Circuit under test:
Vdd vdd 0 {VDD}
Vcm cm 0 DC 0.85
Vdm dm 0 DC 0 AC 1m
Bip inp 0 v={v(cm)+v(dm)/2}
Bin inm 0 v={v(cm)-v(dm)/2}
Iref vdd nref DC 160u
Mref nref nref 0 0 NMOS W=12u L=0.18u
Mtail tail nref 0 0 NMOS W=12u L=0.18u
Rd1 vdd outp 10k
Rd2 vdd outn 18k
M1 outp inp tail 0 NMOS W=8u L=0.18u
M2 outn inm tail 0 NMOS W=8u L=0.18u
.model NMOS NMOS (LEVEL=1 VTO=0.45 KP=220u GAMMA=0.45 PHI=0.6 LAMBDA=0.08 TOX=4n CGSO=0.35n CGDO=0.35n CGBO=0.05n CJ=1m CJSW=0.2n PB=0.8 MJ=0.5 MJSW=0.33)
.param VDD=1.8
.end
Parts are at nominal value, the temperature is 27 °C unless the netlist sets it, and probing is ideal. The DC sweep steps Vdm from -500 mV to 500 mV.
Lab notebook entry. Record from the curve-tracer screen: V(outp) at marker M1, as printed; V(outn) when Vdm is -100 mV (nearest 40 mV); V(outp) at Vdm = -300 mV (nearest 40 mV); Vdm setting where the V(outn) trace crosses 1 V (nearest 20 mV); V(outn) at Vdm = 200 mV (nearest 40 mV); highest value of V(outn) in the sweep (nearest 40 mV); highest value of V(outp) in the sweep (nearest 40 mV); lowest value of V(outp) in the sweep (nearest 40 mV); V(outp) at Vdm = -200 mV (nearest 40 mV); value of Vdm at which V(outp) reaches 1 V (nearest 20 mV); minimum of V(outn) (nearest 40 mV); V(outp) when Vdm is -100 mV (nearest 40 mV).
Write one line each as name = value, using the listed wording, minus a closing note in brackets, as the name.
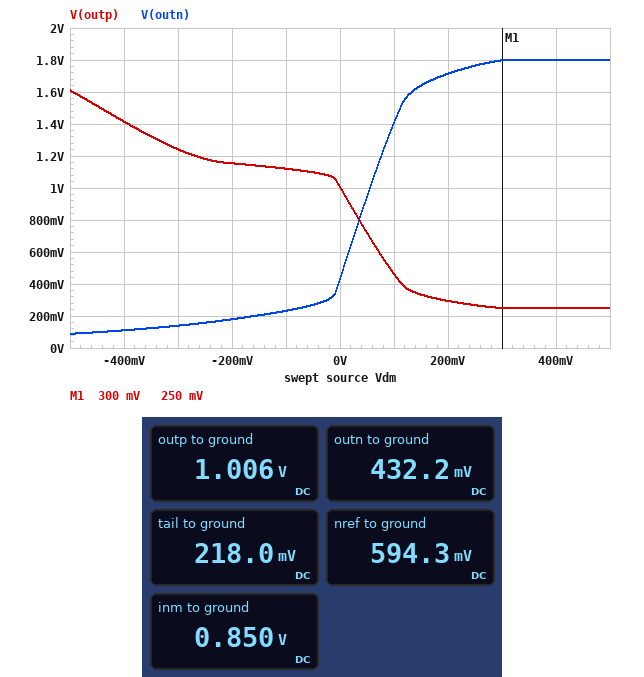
V(outp) at marker M1, as printed = 250 mV
V(outn) when Vdm is -100 mV = 240 mV
V(outp) at Vdm = -300 mV = 1.24 V
Vdm setting where the V(outn) trace crosses 1 V = 60 mV
V(outn) at Vdm = 200 mV = 1.72 V
highest value of V(outn) in the sweep = 1.80 V
highest value of V(outp) in the sweep = 1.60 V
lowest value of V(outp) in the sweep = 240 mV
V(outp) at Vdm = -200 mV = 1.16 V
value of Vdm at which V(outp) reaches 1 V = 0 V
minimum of V(outn) = 80 mV
V(outp) when Vdm is -100 mV = 1.12 V
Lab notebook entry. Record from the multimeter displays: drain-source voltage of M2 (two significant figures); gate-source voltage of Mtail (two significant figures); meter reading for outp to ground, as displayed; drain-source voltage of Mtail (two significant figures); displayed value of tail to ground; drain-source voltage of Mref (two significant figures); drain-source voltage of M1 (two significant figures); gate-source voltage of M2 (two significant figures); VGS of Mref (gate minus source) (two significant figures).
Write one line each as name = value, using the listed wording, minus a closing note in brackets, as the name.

drain-source voltage of M2 = 210 mV
gate-source voltage of Mtail = 590 mV
meter reading for outp to ground, as displayed = 1.006 V
drain-source voltage of Mtail = 220 mV
displayed value of tail to ground = 218.0 mV
drain-source voltage of Mref = 590 mV
drain-source voltage of M1 = 790 mV
gate-source voltage of M2 = 630 mV
VGS of Mref (gate minus source) = 590 mV
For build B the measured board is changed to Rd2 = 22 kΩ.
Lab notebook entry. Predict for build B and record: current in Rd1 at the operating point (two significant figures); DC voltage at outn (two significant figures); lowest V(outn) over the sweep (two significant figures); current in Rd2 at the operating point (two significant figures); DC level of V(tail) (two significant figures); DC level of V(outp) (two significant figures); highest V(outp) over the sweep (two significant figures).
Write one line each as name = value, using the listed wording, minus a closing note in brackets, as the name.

current in Rd1 at the operating point = 87 µA
DC voltage at outn = 290 mV
lowest V(outn) over the sweep = 77 mV
current in Rd2 at the operating point = 69 µA
DC level of V(tail) = 210 mV
DC level of V(outp) = 930 mV
highest V(outp) over the sweep = 1.5 V
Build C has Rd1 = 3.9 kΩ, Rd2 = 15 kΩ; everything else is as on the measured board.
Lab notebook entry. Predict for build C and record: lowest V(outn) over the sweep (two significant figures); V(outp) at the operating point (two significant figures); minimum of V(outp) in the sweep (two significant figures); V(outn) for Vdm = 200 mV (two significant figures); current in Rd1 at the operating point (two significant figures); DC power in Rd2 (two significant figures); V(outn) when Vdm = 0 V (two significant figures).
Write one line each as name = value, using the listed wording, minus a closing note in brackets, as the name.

lowest V(outn) over the sweep = 100 mV
V(outp) at the operating point = 1.5 V
minimum of V(outp) in the sweep = 1.2 V
V(outn) for Vdm = 200 mV = 1.8 V
current in Rd1 at the operating point = 80 µA
DC power in Rd2 = 85 µW
V(outn) when Vdm = 0 V = 670 mV
